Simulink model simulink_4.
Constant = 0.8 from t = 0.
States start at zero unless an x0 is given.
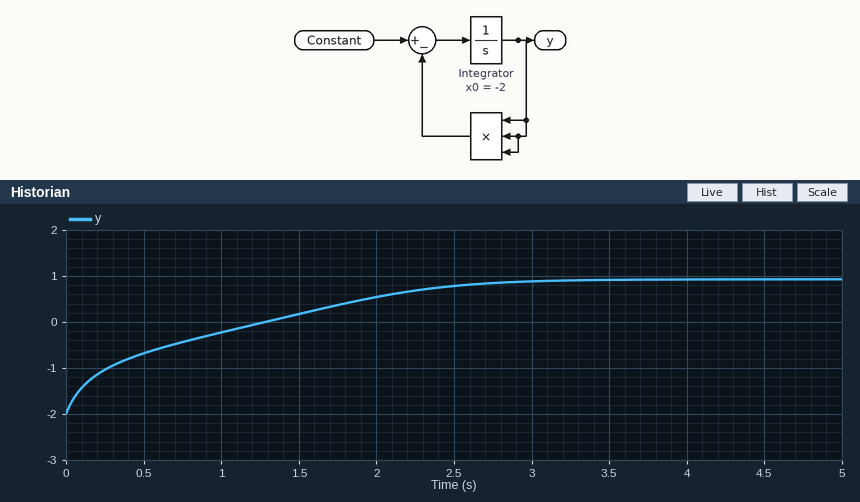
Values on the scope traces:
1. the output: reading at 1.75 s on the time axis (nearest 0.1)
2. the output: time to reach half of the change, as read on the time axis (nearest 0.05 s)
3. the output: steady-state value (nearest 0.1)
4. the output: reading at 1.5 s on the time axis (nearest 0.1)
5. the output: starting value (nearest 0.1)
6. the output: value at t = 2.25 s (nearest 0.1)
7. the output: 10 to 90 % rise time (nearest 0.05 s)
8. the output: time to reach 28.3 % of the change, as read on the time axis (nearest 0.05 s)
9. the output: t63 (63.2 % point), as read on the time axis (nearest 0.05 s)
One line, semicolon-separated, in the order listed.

0.4; 0.65 s; 0.9; 0.2; -2.0; 0.7; 2.10 s; 0.20 s; 1.10 s
